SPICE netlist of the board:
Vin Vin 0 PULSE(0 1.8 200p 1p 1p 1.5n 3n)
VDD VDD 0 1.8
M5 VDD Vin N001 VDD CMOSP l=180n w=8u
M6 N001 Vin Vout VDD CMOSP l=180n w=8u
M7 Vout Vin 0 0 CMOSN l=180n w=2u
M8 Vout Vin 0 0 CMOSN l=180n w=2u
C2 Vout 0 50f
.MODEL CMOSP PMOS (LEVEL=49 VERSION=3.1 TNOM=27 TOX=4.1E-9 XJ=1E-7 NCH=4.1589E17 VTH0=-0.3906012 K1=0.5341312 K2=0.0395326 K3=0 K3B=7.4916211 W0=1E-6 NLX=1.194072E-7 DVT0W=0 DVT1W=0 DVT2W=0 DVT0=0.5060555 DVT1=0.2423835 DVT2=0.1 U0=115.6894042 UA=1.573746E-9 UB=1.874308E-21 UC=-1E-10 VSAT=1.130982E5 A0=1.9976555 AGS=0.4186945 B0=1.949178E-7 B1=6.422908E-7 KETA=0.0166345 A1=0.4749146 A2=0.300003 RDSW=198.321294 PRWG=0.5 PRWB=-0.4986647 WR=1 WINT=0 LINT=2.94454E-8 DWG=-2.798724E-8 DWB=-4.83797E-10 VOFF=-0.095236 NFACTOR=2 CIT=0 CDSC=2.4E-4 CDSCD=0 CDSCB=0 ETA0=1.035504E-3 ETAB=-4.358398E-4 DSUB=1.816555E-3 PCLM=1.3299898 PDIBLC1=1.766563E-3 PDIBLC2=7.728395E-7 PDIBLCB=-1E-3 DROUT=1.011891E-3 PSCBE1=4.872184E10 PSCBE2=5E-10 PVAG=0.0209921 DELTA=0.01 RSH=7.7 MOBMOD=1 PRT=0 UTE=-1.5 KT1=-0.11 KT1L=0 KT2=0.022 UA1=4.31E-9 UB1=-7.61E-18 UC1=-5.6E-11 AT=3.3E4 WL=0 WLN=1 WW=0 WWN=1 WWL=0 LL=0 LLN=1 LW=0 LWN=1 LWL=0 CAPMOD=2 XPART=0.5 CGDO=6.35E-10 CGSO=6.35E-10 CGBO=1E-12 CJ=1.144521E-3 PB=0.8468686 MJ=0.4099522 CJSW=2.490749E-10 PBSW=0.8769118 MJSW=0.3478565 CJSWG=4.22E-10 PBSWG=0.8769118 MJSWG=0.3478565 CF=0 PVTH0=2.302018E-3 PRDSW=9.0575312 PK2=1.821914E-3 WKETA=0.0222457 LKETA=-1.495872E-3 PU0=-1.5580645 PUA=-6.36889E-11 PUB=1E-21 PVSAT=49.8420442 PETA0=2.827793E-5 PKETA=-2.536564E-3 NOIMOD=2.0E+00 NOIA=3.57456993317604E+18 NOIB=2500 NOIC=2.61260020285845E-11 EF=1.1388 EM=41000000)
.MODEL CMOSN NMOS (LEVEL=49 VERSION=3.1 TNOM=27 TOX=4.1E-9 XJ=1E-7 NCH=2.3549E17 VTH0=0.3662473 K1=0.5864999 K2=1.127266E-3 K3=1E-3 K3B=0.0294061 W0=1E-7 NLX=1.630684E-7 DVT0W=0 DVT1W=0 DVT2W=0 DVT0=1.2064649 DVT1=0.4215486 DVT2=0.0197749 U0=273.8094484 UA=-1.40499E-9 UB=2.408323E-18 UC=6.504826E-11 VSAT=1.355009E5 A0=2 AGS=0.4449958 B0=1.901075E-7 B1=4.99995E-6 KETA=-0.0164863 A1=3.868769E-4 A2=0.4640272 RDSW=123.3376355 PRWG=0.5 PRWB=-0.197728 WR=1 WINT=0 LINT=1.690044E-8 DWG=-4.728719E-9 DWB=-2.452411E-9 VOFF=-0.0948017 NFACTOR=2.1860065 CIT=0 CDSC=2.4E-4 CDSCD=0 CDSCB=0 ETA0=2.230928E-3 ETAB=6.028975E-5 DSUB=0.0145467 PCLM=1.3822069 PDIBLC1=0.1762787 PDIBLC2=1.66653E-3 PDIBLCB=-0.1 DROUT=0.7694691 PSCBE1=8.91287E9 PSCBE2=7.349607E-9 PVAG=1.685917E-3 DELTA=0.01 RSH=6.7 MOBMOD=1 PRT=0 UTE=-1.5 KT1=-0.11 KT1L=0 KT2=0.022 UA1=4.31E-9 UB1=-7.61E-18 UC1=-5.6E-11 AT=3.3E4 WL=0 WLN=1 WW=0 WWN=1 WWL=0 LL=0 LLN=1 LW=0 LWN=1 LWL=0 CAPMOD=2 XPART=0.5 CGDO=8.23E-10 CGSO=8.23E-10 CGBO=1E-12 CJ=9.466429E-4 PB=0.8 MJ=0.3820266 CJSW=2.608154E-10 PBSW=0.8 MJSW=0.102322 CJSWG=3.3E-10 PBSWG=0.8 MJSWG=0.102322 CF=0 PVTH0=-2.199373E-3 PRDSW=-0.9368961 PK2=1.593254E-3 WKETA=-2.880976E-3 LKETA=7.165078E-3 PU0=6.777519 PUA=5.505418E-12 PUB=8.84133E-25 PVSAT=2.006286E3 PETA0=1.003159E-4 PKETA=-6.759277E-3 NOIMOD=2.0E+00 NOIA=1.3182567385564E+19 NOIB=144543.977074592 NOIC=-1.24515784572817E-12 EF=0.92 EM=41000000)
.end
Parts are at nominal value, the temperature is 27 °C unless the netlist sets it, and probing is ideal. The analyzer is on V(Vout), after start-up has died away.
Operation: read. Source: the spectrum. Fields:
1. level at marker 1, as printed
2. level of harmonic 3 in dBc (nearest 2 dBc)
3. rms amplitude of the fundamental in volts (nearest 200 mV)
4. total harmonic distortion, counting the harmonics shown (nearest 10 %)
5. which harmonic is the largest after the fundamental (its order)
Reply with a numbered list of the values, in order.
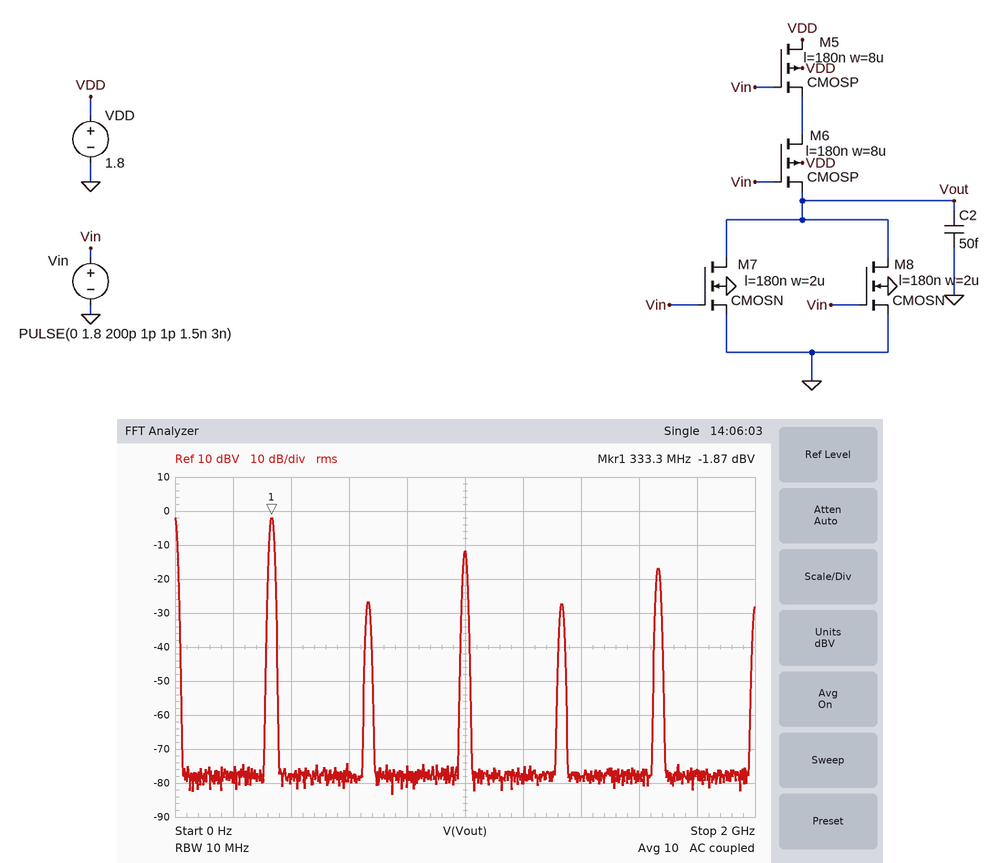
1. -1.87 dBV
2. -10 dBc
3. 800 mV
4. 40 %
5. 3
